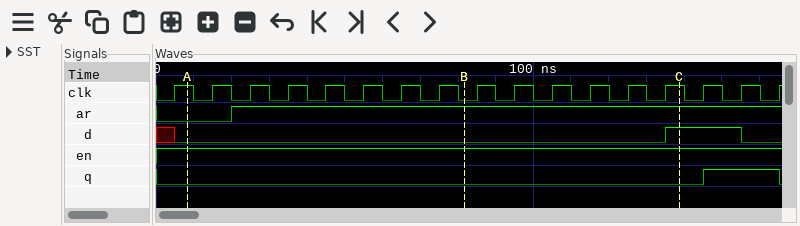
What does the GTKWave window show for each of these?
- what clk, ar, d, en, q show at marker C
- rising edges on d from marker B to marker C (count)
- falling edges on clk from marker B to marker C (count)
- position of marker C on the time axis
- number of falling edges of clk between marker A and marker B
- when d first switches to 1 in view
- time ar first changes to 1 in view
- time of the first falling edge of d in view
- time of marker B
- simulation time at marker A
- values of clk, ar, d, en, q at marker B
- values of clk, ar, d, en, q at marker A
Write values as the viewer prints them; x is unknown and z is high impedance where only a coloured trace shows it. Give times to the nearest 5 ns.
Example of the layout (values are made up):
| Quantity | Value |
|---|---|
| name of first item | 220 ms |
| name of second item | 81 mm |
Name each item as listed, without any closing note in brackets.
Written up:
| Quantity | Value |
|---|---|
| what clk, ar, d, en, q show at marker C | clk=1, ar=1, d=1, en=1, q=0 |
| rising edges on d from marker B to marker C | 1 |
| falling edges on clk from marker B to marker C | 5 |
| position of marker C on the time axis | 140 ns |
| number of falling edges of clk between marker A and marker B | 8 |
| when d first switches to 1 in view | 135 ns |
| time ar first changes to 1 in view | 20 ns |
| time of the first falling edge of d in view | 155 ns |
| time of marker B | 80 ns |
| simulation time at marker A | 10 ns |
| values of clk, ar, d, en, q at marker B | clk=0, ar=1, d=0, en=1, q=0 |
| values of clk, ar, d, en, q at marker A | clk=1, ar=0, d=0, en=1, q=0 |
